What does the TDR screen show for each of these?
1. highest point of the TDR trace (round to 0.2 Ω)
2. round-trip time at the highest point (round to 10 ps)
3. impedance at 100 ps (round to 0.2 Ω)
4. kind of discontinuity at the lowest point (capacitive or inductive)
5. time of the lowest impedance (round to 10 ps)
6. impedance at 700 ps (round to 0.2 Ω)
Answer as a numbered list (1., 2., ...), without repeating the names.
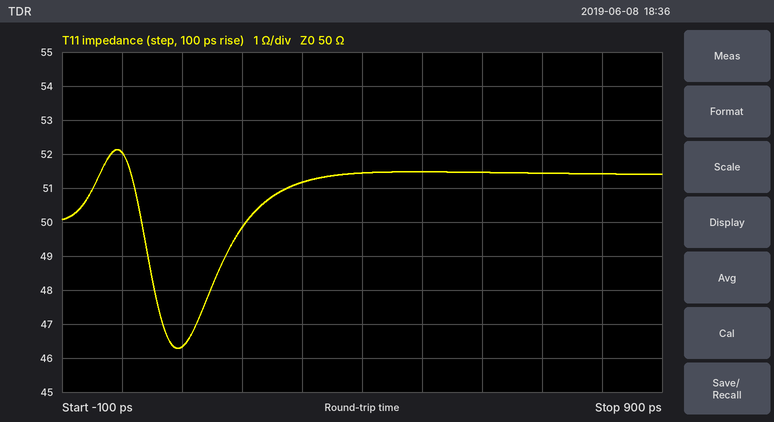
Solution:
1. 52.2 Ω
2. -10 ps
3. 46.4 Ω
4. capacitive
5. 90 ps
6. 51.4 Ω
